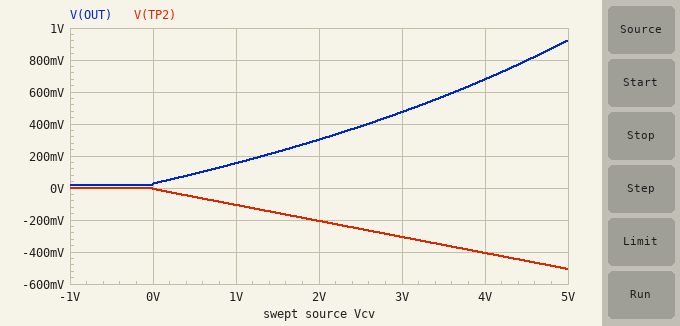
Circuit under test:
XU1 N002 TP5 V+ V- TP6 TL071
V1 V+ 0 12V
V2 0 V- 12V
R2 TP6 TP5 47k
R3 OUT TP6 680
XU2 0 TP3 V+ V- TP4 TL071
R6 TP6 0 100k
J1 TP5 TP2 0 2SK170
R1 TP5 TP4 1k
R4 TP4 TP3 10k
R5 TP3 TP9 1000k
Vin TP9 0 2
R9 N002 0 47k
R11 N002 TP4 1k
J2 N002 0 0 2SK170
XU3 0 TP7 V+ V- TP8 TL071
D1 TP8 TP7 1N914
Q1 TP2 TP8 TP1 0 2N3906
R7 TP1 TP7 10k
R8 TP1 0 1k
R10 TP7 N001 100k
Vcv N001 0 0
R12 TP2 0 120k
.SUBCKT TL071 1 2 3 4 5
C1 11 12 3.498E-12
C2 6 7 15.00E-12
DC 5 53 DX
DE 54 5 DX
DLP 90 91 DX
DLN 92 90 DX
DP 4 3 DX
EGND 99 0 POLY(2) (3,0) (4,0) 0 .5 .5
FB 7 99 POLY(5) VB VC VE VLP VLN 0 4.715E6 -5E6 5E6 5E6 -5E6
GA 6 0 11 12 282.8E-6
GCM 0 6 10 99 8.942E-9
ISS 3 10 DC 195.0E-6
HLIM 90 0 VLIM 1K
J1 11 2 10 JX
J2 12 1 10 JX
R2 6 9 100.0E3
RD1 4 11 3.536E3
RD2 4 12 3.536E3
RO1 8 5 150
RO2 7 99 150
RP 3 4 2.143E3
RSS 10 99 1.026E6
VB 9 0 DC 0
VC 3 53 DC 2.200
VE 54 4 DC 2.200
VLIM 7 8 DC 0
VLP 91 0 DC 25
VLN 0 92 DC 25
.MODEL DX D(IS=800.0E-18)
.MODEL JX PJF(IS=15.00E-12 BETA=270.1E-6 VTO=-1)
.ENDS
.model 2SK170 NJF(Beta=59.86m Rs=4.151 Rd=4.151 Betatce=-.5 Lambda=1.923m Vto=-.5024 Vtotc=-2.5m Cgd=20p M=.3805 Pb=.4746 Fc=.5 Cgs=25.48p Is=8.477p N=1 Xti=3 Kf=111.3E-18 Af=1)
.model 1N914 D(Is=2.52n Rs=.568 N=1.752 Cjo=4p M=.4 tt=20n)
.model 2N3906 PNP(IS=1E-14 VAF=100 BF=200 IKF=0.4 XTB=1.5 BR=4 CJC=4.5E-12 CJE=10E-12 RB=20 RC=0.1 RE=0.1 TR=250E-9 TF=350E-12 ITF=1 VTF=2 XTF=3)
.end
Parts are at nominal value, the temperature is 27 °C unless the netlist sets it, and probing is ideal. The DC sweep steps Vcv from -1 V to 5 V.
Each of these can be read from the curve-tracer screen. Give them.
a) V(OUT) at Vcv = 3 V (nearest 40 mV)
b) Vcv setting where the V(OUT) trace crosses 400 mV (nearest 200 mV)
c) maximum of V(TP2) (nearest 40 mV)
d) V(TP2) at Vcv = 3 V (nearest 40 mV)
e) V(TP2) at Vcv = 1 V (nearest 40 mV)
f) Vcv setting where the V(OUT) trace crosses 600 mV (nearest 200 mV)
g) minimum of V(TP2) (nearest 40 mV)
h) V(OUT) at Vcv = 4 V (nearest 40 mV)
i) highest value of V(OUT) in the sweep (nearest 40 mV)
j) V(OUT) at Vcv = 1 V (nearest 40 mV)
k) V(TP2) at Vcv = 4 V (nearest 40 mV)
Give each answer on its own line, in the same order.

480 mV
2.6 V
0 V
-320 mV
-120 mV
3.6 V
-520 mV
680 mV
920 mV
160 mV
-400 mV
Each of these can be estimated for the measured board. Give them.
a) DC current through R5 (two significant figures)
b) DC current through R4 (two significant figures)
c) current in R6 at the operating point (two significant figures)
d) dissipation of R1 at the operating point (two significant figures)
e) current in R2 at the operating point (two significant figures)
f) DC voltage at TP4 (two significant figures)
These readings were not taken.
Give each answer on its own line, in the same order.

2.0 µA
2.0 µA
210 nA
380 nW
460 nA
-20 mV
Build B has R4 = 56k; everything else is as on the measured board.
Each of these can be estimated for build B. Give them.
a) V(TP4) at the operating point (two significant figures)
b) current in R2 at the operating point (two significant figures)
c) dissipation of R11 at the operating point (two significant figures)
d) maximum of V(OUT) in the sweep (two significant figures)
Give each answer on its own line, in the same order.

-110 mV
510 nA
12 µW
5.1 V
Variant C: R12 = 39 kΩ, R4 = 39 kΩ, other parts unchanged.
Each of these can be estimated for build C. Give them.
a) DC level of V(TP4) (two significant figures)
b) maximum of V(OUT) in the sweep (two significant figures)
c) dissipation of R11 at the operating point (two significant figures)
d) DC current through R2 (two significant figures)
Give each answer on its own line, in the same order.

-78 mV
3.6 V
5.8 µW
490 nA
